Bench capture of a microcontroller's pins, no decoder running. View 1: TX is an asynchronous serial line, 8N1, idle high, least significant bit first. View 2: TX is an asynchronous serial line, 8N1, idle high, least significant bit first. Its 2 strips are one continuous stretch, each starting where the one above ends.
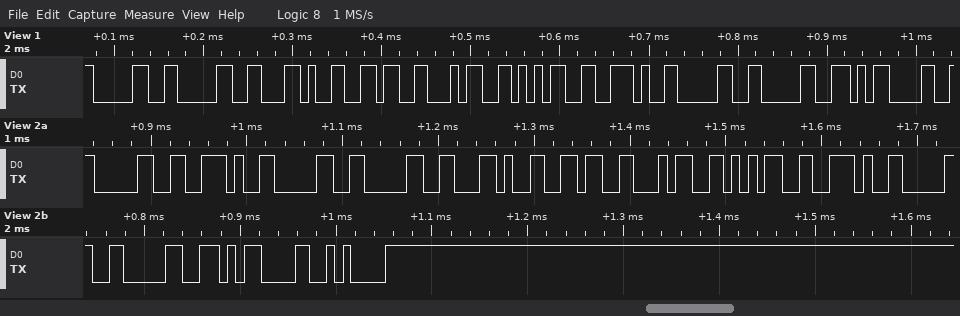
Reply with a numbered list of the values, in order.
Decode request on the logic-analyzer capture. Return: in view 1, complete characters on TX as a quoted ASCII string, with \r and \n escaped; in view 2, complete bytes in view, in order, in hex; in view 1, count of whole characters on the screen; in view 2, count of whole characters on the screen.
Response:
1. "00,645.00\r"
2. 30 2E 30 30 2C 36 34 35 2E 30 30 0D 0A
3. 10
4. 13
